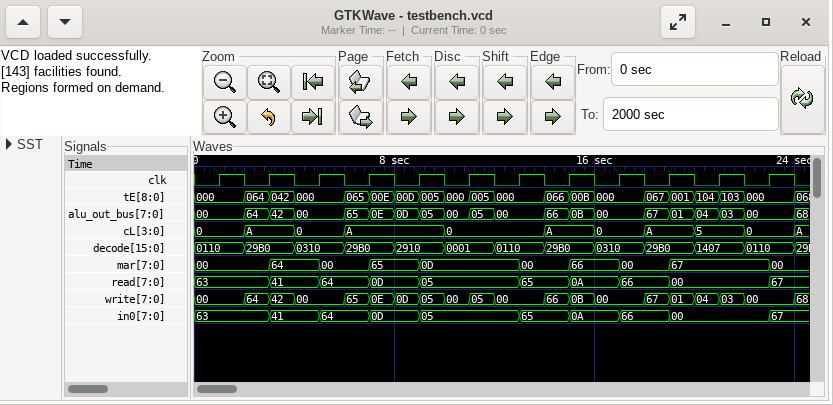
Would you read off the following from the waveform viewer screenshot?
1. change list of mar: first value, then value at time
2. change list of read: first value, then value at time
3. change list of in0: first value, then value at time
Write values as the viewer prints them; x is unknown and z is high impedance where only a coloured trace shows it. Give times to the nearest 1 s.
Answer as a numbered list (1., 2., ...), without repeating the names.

1. 00, 64 at 3 s, 00 at 5 s, 65 at 7 s, 0D at 9 s, 00 at 13 s, 66 at 15 s, 00 at 17 s, 67 at 19 s, 00 at 23 s
2. 63, 41 at 3 s, 64 at 5 s, 0D at 7 s, 05 at 9 s, 65 at 13 s, 0A at 15 s, 66 at 17 s, 00 at 19 s, 67 at 23 s
3. 63, 41 at 3 s, 64 at 5 s, 0D at 7 s, 05 at 9 s, 65 at 13 s, 0A at 15 s, 66 at 17 s, 00 at 19 s, 67 at 23 s
